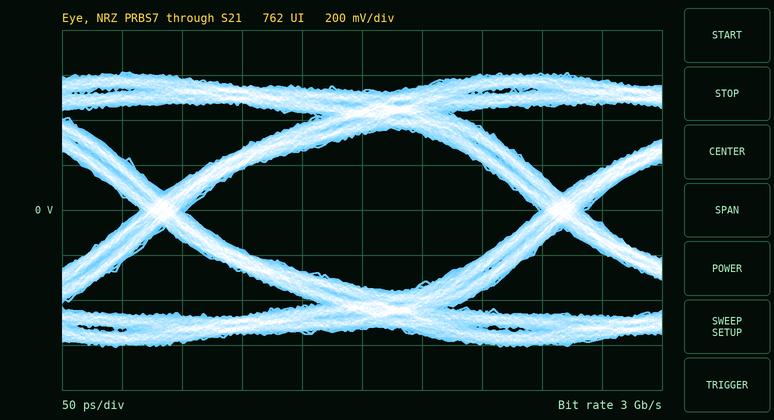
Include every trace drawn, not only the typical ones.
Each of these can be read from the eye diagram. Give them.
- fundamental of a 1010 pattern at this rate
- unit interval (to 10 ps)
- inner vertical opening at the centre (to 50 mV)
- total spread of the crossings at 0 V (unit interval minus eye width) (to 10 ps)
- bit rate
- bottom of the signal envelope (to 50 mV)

1.5 GHz
330 ps
700 mV
40 ps
3 Gb/s
-600 mV
